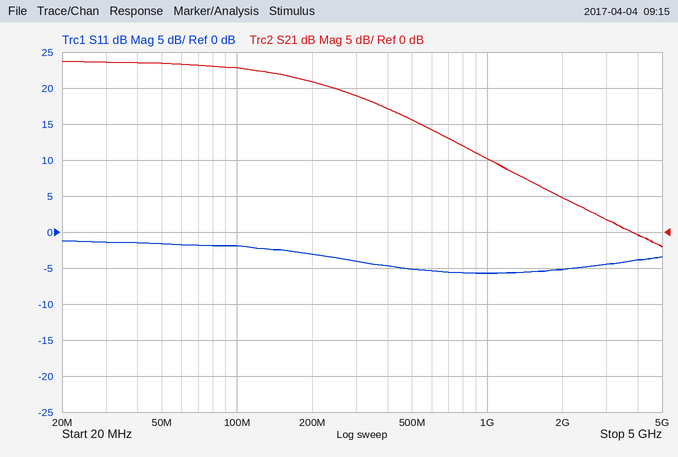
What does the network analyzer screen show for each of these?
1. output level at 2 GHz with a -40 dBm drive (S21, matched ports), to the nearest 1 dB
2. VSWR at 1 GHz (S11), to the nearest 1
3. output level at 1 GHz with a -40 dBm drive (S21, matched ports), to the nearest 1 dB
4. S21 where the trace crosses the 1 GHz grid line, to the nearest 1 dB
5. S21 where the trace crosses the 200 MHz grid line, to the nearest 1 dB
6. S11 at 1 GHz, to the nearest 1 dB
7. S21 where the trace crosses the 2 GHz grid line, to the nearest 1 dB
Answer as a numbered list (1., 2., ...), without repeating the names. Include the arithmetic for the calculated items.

1. -40 dBm + (5 dB) = -35 dBm
2. |Γ| = 10^(-6/20) = 0.5012; VSWR = (1 + 0.5012)/(1 − 0.5012) ≈ 3
3. -40 dBm + (10 dB) = -30 dBm
4. 10 dB
5. 21 dB
6. -6 dB
7. 5 dB
